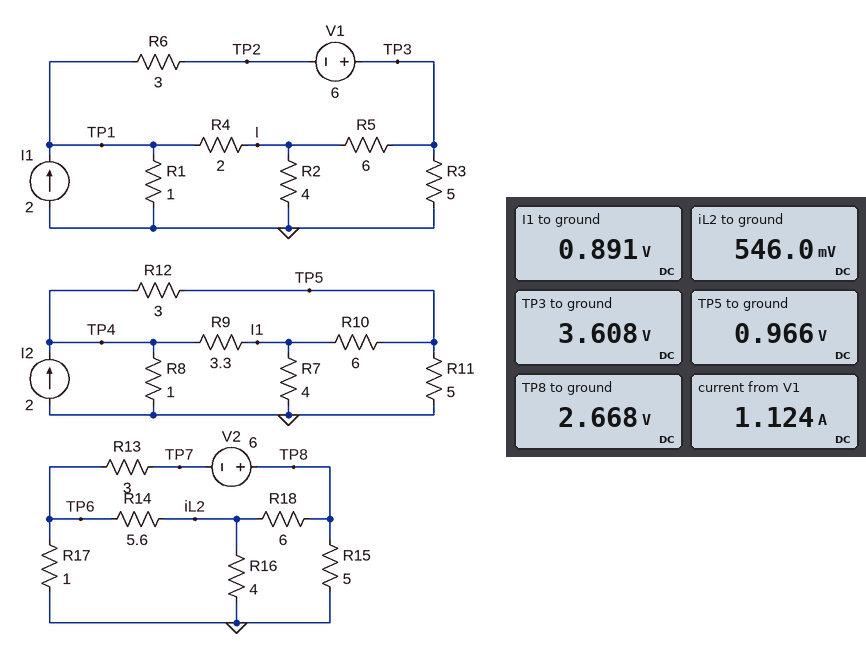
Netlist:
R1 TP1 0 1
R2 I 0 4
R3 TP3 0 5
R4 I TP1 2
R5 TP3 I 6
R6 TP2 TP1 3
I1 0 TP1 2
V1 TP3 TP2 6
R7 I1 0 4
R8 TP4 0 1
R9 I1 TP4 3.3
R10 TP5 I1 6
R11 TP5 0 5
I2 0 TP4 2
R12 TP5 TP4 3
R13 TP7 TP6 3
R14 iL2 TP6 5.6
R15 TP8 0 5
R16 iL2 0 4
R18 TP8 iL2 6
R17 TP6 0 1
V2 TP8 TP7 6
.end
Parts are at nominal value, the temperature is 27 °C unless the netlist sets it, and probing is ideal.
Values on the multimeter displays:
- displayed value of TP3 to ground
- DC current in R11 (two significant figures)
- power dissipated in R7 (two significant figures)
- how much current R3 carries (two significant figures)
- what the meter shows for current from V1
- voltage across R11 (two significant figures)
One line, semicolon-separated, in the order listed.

3.608 V; 190 mA; 200 mW; 720 mA; 1.124 A; 970 mV
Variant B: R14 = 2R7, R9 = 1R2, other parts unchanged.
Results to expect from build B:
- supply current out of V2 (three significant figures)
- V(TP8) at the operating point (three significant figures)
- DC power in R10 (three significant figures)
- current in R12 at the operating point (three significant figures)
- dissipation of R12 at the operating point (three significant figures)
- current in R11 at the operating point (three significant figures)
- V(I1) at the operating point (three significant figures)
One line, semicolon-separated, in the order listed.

921 mA; 2.64 V; 3.70 mW; 174 mA; 90.7 mW; 199 mA; 1.14 V
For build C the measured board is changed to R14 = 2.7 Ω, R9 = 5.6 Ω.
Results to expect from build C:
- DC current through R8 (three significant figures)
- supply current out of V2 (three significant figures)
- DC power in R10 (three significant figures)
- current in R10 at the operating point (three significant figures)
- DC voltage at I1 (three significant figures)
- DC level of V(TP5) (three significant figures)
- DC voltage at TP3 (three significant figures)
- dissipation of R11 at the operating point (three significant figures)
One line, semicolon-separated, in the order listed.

1.62 A; 921 mA; 6.57 mW; 33.1 mA; 753 mV; 951 mV; 3.61 V; 181 mW
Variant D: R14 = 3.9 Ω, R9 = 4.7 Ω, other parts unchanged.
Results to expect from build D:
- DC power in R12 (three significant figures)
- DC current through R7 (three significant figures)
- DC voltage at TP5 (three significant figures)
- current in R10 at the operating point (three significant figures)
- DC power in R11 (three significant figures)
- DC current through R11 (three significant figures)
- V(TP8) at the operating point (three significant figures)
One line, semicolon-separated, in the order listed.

142 mW; 199 mA; 956 mV; 26.5 mA; 183 mW; 191 mA; 2.65 V
